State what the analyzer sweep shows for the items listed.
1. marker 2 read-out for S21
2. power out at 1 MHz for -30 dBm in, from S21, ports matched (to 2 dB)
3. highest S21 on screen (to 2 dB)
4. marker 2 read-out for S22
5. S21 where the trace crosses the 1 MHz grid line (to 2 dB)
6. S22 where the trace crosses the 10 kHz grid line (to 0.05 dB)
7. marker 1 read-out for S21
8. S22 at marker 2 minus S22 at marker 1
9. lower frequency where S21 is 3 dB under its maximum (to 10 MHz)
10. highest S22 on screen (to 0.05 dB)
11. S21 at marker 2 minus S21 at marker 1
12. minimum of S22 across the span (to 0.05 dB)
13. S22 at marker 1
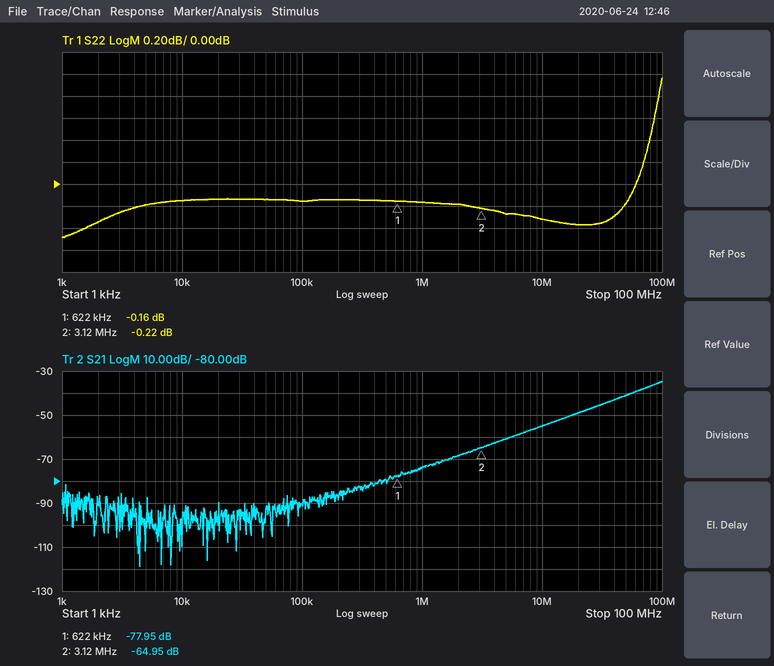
-64.95 dB
-104 dBm
-34 dB
-0.22 dB
-74 dB
-0.15 dB
-77.95 dB
-0.06 dB
70 MHz
0.95 dB
13.00 dB
-0.50 dB
-0.16 dB
